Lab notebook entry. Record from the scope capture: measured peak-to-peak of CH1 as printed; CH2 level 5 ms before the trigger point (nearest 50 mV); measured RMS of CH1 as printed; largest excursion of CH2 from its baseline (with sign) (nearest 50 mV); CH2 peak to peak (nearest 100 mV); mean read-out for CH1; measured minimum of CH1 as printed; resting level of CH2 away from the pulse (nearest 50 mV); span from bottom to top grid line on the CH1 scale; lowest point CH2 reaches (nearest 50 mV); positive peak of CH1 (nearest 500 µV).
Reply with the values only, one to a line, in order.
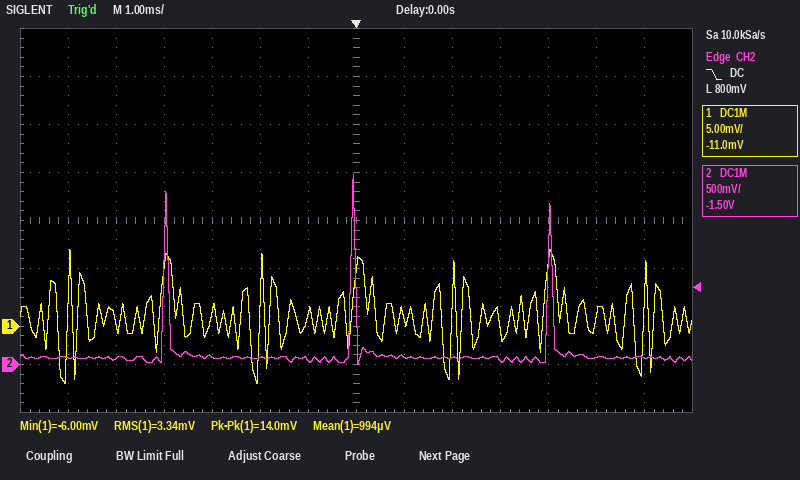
14.0 mV
50 mV
3.34 mV
+1.90 V
2.00 V
994 µV
-6.00 mV
50 mV
40 mV
0 mV
8.0 mV
